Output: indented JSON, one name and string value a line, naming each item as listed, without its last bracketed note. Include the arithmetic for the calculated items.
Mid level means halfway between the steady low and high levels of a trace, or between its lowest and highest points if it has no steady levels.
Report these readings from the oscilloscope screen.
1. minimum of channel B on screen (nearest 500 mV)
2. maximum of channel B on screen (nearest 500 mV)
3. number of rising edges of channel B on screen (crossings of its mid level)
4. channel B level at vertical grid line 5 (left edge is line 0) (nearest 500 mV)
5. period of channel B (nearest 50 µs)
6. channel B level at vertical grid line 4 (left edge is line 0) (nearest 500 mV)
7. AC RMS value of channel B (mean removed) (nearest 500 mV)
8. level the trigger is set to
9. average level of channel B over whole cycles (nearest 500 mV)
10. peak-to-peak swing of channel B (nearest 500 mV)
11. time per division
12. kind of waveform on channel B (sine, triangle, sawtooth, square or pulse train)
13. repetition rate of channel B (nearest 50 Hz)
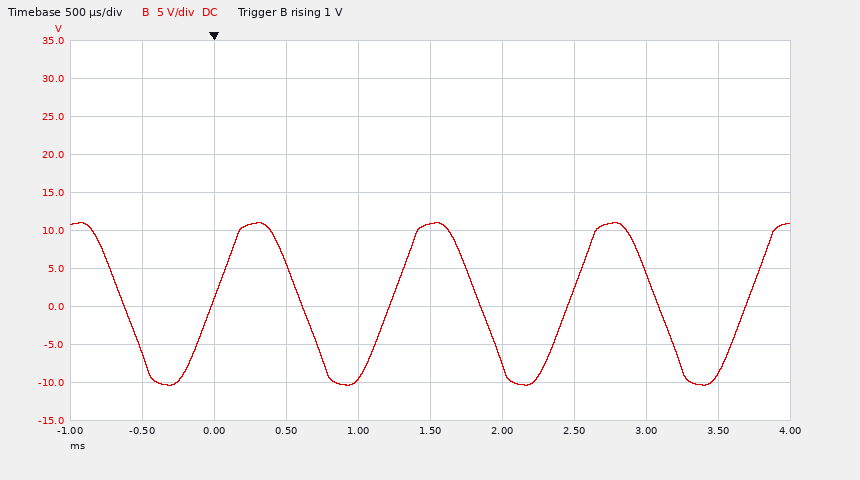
{
  "minimum of channel B on screen": "-10.5 V",
  "maximum of channel B on screen": "11.0 V",
  "number of rising edges of channel B on screen": "4",
  "channel B level at vertical grid line 5 (left edge is line 0)": "11.0 V",
  "period of channel B": "1.25 ms",
  "channel B level at vertical grid line 4 (left edge is line 0)": "-9.5 V",
  "AC RMS value of channel B (mean removed)": "21.5 V / (2√2) ≈ 7.60 V, so 7.5 V to the nearest 500 mV",
  "level the trigger is set to": "1 V",
  "average level of channel B over whole cycles": "(11.0 V + (-10.5 V)) / 2 ≈ 250 mV, so 500 mV to the nearest 500 mV",
  "peak-to-peak swing of channel B": "11.0 V − (-10.5 V) = 21.5 V",
  "time per division": "500 µs",
  "kind of waveform on channel B": "sine",
  "repetition rate of channel B": "1 / 1.25 ms ≈ 800 Hz"
}
